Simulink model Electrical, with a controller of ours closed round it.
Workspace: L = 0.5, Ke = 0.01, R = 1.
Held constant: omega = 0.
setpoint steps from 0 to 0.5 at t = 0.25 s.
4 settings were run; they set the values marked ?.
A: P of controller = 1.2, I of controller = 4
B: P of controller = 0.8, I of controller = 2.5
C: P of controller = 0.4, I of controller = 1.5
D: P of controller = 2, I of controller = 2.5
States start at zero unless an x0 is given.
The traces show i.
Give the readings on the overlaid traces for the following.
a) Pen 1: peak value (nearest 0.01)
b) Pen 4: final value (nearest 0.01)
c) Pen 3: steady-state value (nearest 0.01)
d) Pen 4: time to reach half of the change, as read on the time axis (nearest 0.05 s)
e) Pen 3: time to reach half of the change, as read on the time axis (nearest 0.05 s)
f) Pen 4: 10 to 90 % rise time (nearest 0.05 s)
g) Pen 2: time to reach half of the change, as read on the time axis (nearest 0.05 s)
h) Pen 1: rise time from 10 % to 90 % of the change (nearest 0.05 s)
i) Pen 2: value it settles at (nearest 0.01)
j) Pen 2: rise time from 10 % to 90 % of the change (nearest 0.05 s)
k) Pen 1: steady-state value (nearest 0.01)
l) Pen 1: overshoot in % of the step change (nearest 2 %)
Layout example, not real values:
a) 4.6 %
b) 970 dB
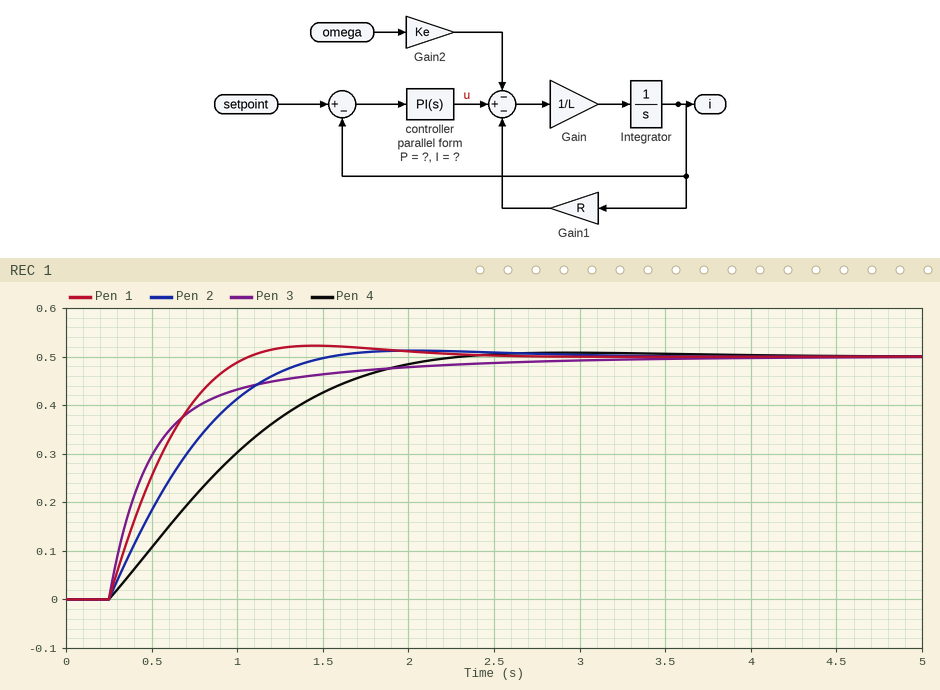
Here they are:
a) 0.52
b) 0.50
c) 0.50
d) 0.85 s
e) 0.45 s
f) 1.30 s
g) 0.60 s
h) 0.55 s
i) 0.50
j) 0.85 s
k) 0.50
l) 4 %
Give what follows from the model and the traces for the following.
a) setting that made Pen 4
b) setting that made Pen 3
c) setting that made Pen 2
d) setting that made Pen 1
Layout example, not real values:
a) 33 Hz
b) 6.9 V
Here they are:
a) C
b) D
c) B
d) A
